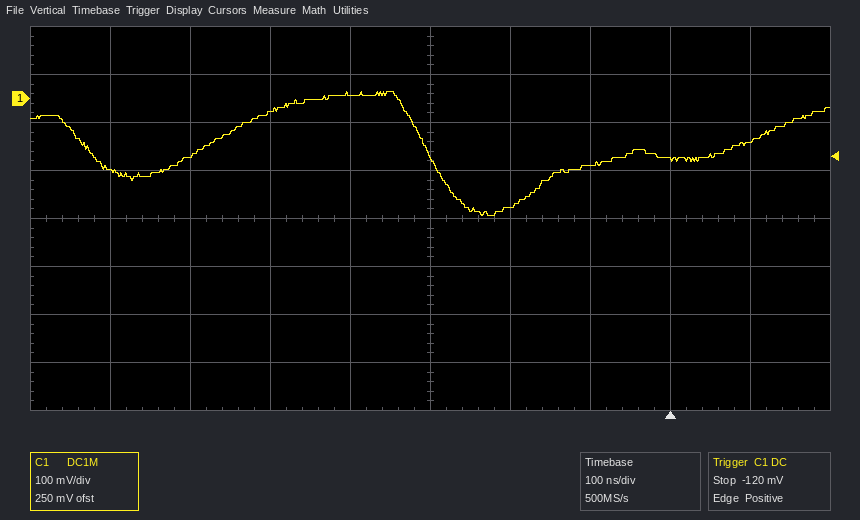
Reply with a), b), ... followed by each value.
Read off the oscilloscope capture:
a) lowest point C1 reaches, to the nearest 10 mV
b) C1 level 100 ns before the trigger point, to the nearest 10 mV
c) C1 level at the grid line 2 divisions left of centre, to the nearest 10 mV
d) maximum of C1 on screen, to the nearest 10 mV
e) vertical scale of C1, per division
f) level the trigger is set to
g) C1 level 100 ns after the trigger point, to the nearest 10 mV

a) -240 mV
b) -140 mV
c) -30 mV
d) 10 mV
e) 100 mV
f) -120 mV
g) -90 mV
